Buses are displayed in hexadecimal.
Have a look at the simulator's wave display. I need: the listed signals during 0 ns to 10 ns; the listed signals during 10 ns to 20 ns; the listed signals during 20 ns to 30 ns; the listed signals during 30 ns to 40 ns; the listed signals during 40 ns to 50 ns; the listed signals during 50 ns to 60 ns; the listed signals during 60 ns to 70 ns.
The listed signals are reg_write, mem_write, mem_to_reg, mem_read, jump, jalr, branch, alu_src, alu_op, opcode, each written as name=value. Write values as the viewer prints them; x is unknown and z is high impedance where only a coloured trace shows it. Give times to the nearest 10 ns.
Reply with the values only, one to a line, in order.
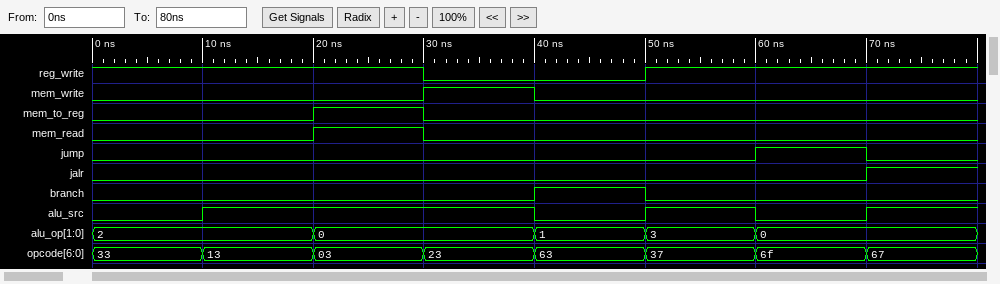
reg_write=1, mem_write=0, mem_to_reg=0, mem_read=0, jump=0, jalr=0, branch=0, alu_src=0, alu_op=2, opcode=33
reg_write=1, mem_write=0, mem_to_reg=0, mem_read=0, jump=0, jalr=0, branch=0, alu_src=1, alu_op=2, opcode=13
reg_write=1, mem_write=0, mem_to_reg=1, mem_read=1, jump=0, jalr=0, branch=0, alu_src=1, alu_op=0, opcode=03
reg_write=0, mem_write=1, mem_to_reg=0, mem_read=0, jump=0, jalr=0, branch=0, alu_src=1, alu_op=0, opcode=23
reg_write=0, mem_write=0, mem_to_reg=0, mem_read=0, jump=0, jalr=0, branch=1, alu_src=0, alu_op=1, opcode=63
reg_write=1, mem_write=0, mem_to_reg=0, mem_read=0, jump=0, jalr=0, branch=0, alu_src=1, alu_op=3, opcode=37
reg_write=1, mem_write=0, mem_to_reg=0, mem_read=0, jump=1, jalr=0, branch=0, alu_src=0, alu_op=0, opcode=6f
